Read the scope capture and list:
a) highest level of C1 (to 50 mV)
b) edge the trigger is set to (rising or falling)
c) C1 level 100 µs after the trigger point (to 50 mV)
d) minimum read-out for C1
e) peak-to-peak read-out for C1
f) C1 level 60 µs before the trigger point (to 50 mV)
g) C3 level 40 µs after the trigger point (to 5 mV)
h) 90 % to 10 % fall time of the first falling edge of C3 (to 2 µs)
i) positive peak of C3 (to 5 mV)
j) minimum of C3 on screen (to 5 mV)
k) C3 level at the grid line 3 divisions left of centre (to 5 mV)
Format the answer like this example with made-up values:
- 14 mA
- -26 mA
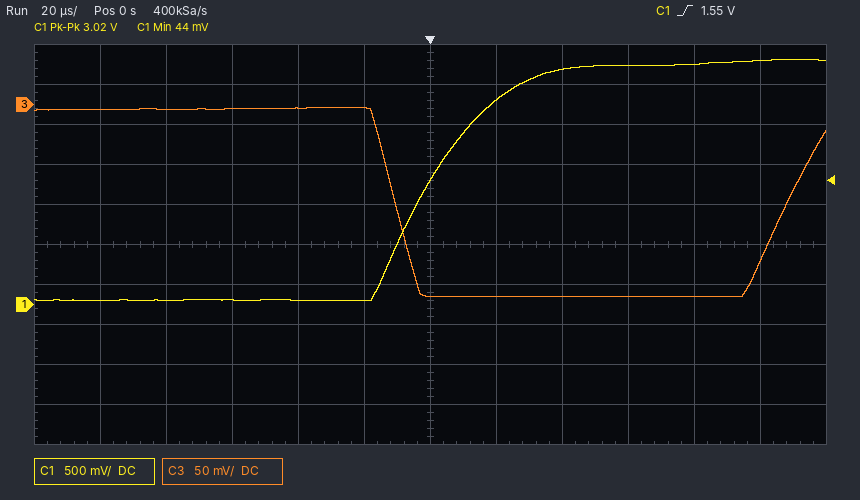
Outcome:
- 3.05 V
- rising
- 3.05 V
- 44 mV
- 3.02 V
- 50 mV
- -240 mV
- 12 µs
- -5 mV
- -240 mV
- -5 mV
